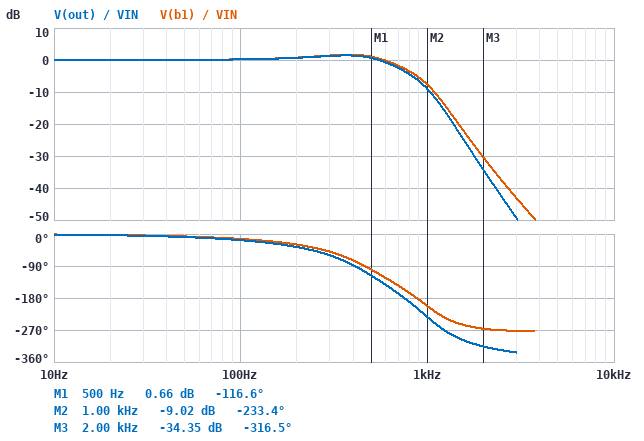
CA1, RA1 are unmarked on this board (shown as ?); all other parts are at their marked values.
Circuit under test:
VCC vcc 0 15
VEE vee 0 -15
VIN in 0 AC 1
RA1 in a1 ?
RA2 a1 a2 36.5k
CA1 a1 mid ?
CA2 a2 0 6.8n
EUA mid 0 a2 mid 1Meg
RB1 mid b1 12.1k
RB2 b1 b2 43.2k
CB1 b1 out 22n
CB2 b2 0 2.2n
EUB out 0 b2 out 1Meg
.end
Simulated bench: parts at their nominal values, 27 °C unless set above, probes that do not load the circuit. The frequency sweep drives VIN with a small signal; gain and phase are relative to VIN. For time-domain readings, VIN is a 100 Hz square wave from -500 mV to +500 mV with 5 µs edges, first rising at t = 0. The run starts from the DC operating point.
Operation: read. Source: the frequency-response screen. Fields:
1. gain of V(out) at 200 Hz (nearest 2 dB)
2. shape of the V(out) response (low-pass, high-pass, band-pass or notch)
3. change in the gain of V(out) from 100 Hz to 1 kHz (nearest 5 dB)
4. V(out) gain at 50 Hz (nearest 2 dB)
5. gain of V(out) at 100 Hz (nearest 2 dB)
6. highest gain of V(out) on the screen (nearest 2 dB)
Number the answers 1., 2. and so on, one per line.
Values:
1. 0 dB
2. low-pass
3. -10 dB
4. 0 dB
5. 0 dB
6. 2 dB
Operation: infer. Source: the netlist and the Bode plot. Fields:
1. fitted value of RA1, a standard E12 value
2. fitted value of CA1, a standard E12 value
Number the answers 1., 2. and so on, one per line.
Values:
1. 15 kΩ
2. 27 nF
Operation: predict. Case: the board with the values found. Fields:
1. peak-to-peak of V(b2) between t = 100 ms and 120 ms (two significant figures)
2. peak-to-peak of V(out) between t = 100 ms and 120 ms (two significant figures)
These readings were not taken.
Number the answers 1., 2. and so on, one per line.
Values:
1. 1.4 V
2. 1.4 V
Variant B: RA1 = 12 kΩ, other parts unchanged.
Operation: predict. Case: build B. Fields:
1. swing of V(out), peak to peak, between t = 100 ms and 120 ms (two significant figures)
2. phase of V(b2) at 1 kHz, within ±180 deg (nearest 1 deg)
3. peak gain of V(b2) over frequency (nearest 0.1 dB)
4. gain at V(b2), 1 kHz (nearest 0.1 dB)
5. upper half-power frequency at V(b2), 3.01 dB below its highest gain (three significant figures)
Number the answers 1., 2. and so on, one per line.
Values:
1. 1.4 V
2. 134 deg
3. 1.3 dB
4. -7.2 dB
5. 733 Hz
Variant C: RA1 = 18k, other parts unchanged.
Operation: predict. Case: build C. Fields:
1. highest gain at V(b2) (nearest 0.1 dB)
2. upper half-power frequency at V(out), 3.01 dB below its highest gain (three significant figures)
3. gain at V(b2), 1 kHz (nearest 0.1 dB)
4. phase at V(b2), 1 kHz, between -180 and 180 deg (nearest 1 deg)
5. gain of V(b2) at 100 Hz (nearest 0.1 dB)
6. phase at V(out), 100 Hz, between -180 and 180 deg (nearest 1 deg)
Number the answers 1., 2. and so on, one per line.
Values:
1. 1.5 dB
2. 582 Hz
3. -10.6 dB
4. 122 deg
5. 0.2 dB
6. -18 deg
